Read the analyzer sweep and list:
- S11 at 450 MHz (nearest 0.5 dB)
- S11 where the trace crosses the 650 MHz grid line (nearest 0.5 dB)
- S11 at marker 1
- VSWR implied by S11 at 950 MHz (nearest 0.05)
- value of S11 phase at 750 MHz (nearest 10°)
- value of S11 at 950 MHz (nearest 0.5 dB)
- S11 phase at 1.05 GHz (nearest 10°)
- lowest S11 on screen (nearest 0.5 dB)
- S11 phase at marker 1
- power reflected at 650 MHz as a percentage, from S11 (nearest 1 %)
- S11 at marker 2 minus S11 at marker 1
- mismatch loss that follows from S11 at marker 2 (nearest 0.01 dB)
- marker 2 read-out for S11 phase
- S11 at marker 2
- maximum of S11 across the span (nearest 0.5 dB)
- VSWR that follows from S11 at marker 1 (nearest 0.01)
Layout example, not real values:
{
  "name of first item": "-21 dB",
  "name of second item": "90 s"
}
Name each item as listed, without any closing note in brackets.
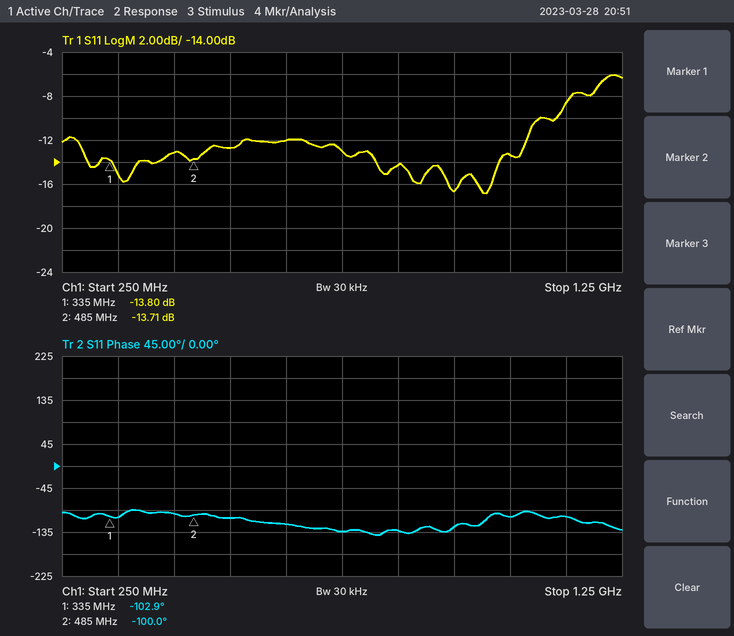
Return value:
{
  "S11 at 450 MHz": "-13.0 dB",
  "S11 where the trace crosses the 650 MHz grid line": "-12.0 dB",
  "S11 at marker 1": "-13.80 dB",
  "VSWR implied by S11 at 950 MHz": "1.35",
  "value of S11 phase at 750 MHz": "-130°",
  "value of S11 at 950 MHz": "-16.5 dB",
  "S11 phase at 1.05 GHz": "-100°",
  "lowest S11 on screen": "-17.0 dB",
  "S11 phase at marker 1": "-102.9°",
  "power reflected at 650 MHz as a percentage, from S11": "6 %",
  "S11 at marker 2 minus S11 at marker 1": "0.09 dB",
  "mismatch loss that follows from S11 at marker 2": "0.19 dB",
  "marker 2 read-out for S11 phase": "-100.0°",
  "S11 at marker 2": "-13.71 dB",
  "maximum of S11 across the span": "-6.0 dB",
  "VSWR that follows from S11 at marker 1": "1.51"
}
